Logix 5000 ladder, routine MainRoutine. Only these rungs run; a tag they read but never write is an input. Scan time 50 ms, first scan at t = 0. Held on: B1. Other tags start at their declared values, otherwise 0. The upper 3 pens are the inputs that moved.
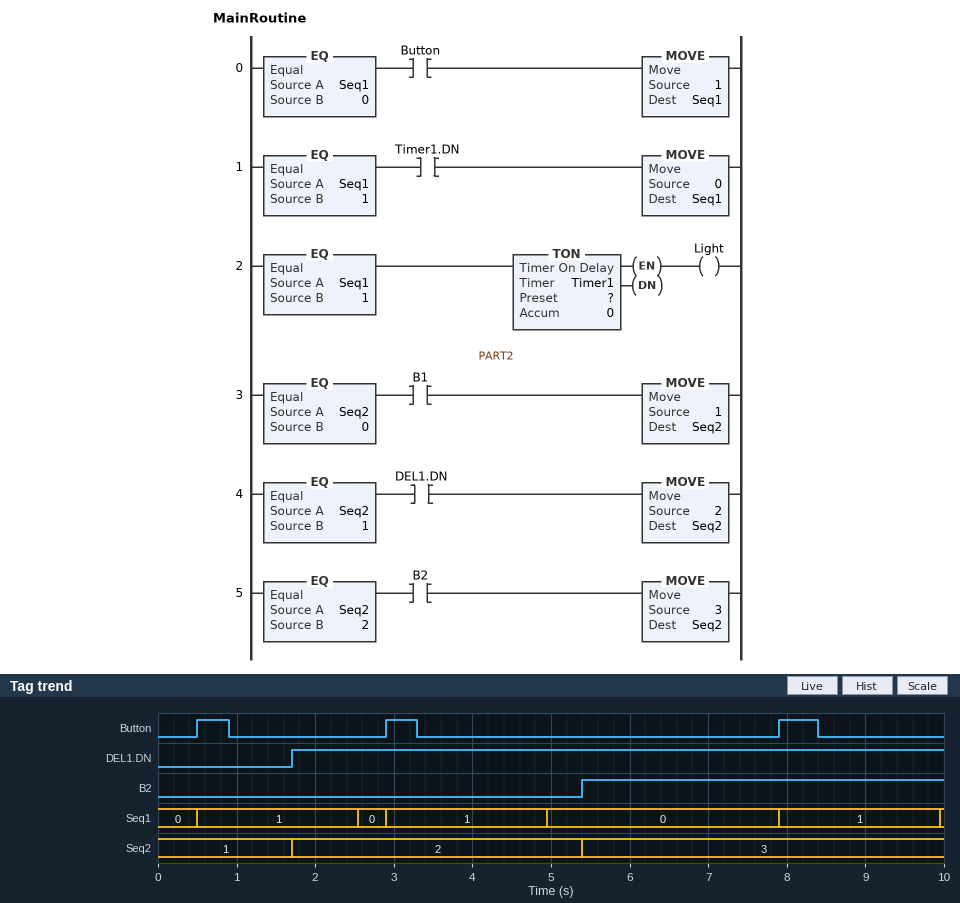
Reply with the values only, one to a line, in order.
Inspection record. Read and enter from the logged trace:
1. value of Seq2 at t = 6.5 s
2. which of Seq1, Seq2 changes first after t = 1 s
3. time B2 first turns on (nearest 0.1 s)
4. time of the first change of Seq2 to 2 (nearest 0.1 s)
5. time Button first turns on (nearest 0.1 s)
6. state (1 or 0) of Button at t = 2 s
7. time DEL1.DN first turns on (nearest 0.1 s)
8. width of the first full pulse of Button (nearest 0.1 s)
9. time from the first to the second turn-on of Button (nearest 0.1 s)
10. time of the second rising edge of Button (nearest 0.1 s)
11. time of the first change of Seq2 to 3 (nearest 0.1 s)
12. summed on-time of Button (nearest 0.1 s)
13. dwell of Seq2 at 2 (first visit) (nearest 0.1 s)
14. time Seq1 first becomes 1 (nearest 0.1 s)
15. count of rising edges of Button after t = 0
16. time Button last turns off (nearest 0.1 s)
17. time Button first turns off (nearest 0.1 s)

3
Seq2
5.4 s
1.7 s
0.5 s
0
1.7 s
0.4 s
2.4 s
2.9 s
5.4 s
1.3 s
3.7 s
0.5 s
3
8.4 s
0.9 s
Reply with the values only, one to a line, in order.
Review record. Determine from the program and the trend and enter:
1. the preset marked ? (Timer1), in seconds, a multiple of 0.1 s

2.0 s
